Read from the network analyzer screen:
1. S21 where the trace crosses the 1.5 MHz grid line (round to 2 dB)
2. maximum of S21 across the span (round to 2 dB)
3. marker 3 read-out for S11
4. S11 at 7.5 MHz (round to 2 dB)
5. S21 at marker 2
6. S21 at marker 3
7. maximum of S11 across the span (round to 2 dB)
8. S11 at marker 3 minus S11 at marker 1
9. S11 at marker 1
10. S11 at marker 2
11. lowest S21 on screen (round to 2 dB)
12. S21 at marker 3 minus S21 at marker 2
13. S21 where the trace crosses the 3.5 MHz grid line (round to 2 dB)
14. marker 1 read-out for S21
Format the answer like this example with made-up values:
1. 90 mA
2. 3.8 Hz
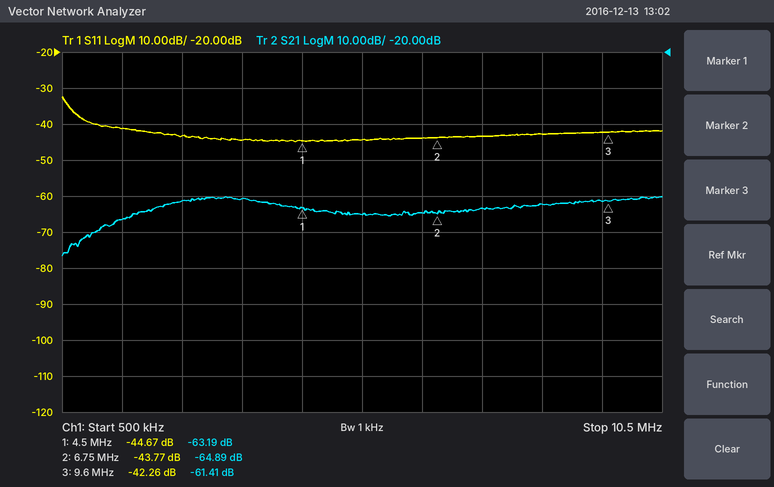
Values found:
1. -66 dB
2. -60 dB
3. -42.26 dB
4. -44 dB
5. -64.89 dB
6. -61.41 dB
7. -32 dB
8. 2.41 dB
9. -44.67 dB
10. -43.77 dB
11. -76 dB
12. 3.48 dB
13. -60 dB
14. -63.19 dB
